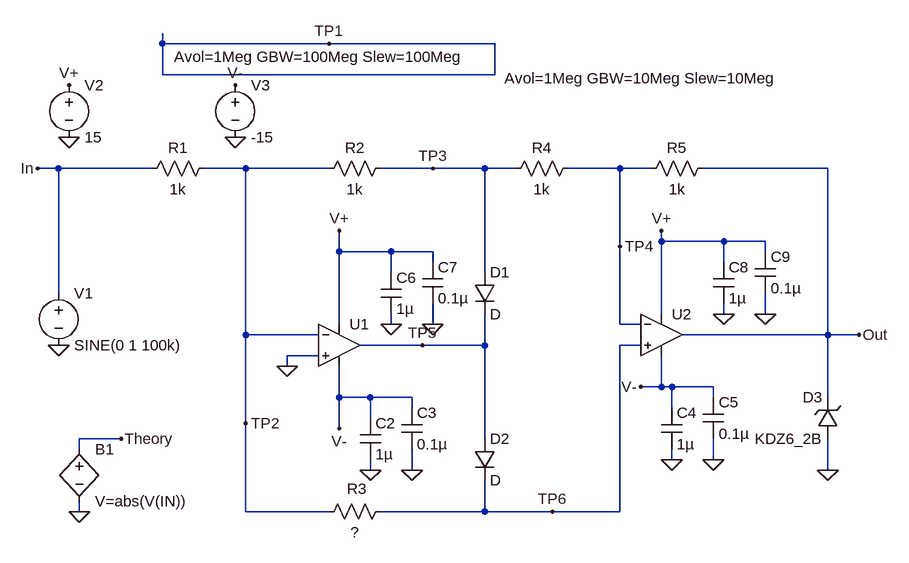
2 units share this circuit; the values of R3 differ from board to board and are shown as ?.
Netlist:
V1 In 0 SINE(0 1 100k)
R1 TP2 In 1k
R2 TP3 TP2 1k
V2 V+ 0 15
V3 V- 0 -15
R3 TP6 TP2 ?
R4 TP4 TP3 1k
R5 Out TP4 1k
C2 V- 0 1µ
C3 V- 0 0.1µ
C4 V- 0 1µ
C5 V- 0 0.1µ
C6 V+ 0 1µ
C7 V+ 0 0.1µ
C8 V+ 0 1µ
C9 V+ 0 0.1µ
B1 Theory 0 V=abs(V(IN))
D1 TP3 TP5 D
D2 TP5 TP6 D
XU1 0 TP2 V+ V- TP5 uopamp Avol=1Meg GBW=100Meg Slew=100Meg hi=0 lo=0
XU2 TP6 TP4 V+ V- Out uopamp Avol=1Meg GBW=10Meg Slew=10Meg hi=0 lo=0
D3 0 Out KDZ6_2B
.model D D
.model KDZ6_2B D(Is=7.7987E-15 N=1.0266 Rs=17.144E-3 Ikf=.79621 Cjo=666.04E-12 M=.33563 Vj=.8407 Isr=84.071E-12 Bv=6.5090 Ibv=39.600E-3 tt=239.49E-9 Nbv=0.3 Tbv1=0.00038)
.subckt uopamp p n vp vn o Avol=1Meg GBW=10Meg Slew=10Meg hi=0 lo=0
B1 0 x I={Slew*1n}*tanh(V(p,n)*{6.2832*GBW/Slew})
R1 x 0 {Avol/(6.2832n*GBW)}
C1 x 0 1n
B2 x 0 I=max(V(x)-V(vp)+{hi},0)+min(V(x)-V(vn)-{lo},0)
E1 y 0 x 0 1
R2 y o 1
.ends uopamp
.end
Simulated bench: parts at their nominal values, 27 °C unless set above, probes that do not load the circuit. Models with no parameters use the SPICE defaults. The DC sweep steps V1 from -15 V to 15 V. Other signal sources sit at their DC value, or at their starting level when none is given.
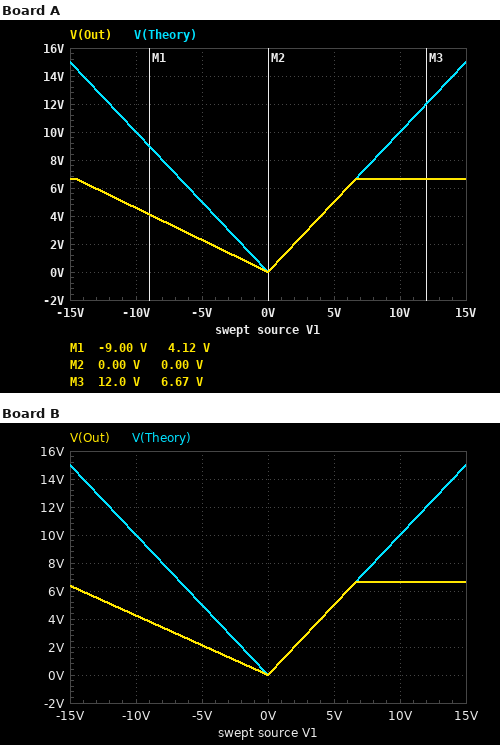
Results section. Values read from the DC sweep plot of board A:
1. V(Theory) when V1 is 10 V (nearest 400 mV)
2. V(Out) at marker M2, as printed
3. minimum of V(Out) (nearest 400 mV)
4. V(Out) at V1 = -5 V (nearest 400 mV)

10.0 V
0.00 V
0 V
2.4 V
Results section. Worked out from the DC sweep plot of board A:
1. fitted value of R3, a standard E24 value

360 Ω
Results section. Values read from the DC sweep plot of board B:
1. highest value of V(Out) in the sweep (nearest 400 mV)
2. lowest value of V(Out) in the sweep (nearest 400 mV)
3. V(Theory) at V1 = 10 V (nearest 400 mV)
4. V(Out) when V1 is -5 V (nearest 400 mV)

6.8 V
0 V
10.0 V
2.0 V
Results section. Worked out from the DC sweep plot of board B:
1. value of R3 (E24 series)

330 Ω
